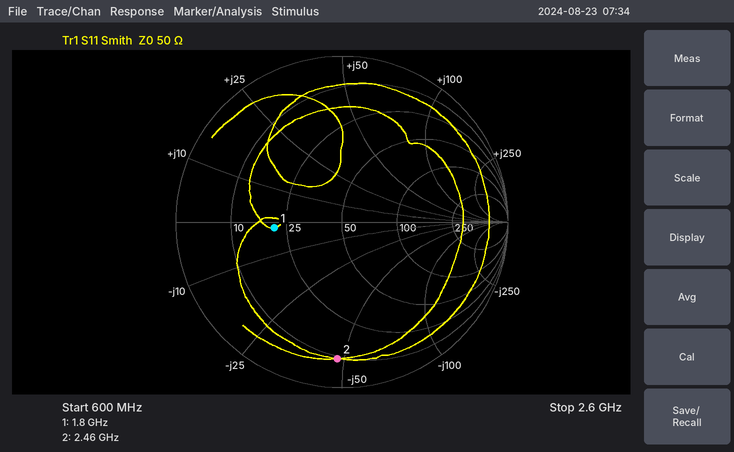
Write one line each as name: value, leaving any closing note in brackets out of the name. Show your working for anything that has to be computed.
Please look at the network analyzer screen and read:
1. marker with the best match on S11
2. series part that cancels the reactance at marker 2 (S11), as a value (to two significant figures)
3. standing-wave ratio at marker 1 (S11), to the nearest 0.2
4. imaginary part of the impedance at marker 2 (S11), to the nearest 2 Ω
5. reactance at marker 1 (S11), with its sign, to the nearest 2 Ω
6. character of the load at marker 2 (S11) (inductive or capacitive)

marker with the best match on S11: marker 1
series part that cancels the reactance at marker 2 (S11), as a value: L = 48 Ω/(2π × 2.46 GHz) ≈ 3.1 nH
standing-wave ratio at marker 1 (S11), to the nearest 0.2: 2.4
imaginary part of the impedance at marker 2 (S11), to the nearest 2 Ω: -48 Ω
reactance at marker 1 (S11), with its sign, to the nearest 2 Ω: -2 Ω
character of the load at marker 2 (S11): capacitive
